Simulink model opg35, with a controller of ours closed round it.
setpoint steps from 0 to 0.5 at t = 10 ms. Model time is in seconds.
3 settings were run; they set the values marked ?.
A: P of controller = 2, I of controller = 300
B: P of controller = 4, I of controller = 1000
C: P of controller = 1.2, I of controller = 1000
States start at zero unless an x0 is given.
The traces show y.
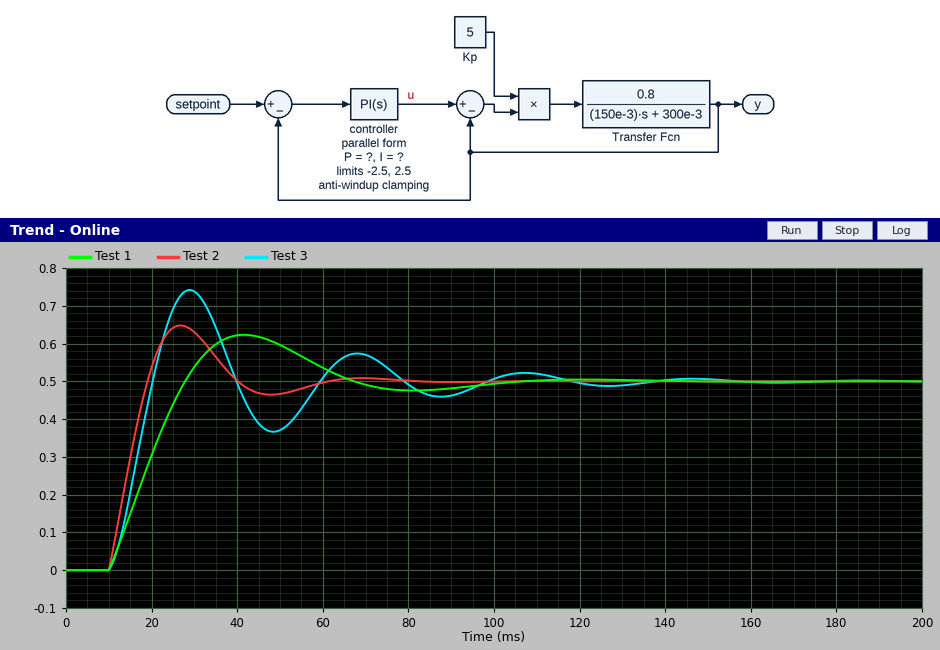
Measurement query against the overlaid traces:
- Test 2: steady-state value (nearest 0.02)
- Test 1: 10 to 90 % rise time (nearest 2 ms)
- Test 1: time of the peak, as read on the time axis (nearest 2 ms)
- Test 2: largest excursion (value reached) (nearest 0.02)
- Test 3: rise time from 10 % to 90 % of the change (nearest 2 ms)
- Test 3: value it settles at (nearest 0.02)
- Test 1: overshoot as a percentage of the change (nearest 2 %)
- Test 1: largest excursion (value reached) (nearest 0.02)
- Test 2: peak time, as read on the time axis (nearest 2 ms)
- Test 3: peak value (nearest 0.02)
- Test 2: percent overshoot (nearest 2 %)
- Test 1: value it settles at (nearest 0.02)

0.50
14 ms
42 ms
0.64
8 ms
0.50
24 %
0.62
26 ms
0.74
30 %
0.50
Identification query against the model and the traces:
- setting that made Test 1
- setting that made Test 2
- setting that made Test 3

A
B
C
